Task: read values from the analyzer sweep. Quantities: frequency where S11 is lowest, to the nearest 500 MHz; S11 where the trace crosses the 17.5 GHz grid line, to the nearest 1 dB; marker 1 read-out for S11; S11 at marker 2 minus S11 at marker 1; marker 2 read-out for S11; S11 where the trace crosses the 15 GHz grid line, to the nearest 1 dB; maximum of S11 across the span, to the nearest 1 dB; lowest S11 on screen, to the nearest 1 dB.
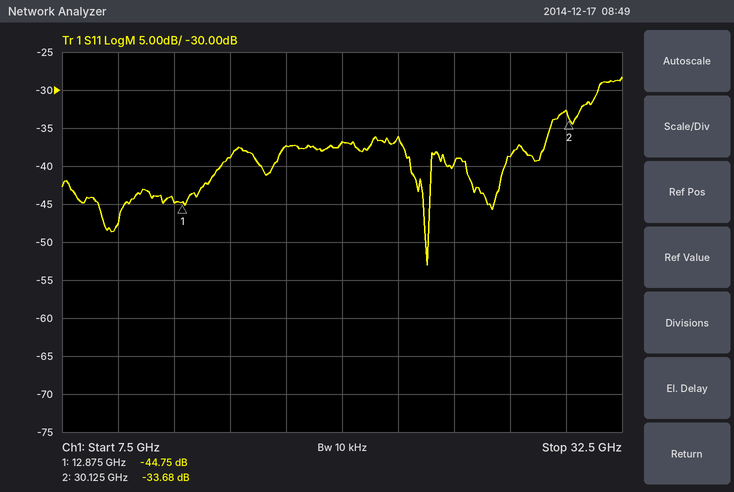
24.0 GHz
-37 dB
-44.75 dB
11.07 dB
-33.68 dB
-39 dB
-28 dB
-53 dB
